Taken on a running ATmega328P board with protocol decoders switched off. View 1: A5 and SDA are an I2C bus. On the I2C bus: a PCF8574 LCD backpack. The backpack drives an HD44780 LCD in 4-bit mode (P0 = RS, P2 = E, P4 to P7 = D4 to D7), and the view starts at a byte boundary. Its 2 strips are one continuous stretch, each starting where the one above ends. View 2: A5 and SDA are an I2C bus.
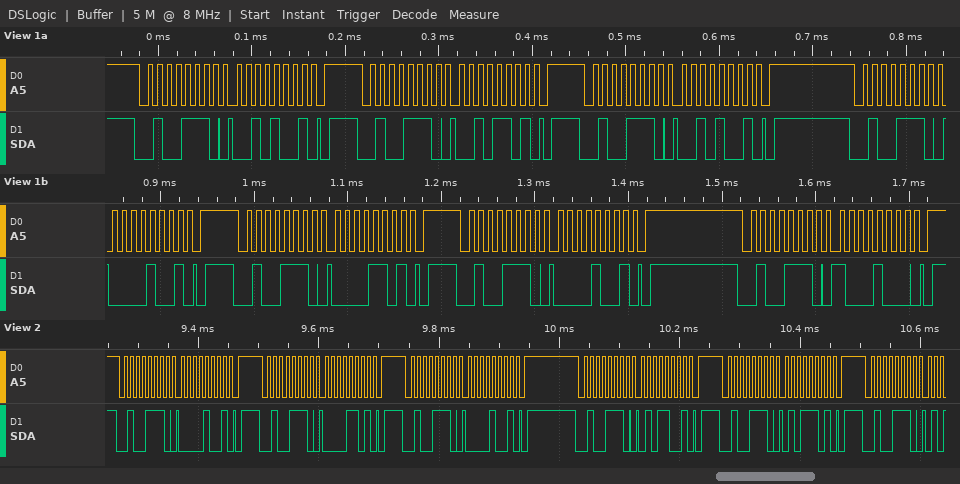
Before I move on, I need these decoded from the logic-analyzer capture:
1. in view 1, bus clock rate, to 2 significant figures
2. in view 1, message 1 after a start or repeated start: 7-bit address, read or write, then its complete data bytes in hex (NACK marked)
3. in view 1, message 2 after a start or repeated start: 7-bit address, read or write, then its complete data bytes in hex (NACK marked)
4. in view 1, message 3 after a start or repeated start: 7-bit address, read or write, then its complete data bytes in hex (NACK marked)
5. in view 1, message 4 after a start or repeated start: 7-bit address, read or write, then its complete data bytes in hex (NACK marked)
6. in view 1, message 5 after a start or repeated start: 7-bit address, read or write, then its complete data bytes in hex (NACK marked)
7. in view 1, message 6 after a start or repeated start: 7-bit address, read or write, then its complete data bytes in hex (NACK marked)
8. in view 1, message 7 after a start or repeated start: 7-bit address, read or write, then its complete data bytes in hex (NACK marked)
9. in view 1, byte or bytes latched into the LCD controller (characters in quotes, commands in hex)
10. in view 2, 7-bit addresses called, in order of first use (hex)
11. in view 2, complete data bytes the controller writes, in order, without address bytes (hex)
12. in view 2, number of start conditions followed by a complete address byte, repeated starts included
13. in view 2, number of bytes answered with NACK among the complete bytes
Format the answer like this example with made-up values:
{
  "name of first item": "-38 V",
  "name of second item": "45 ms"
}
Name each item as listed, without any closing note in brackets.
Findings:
{
  "in view 1, bus clock rate, to 2 significant figures": "100 kHz",
  "in view 1, message 1 after a start or repeated start: 7-bit address, read or write, then its complete data bytes in hex": "0x27 write: 29",
  "in view 1, message 2 after a start or repeated start: 7-bit address, read or write, then its complete data bytes in hex": "0x27 write: 2D",
  "in view 1, message 3 after a start or repeated start: 7-bit address, read or write, then its complete data bytes in hex": "0x27 write: 29",
  "in view 1, message 4 after a start or repeated start: 7-bit address, read or write, then its complete data bytes in hex": "0x27 write: 09",
  "in view 1, message 5 after a start or repeated start: 7-bit address, read or write, then its complete data bytes in hex": "0x27 write: 0D",
  "in view 1, message 6 after a start or repeated start: 7-bit address, read or write, then its complete data bytes in hex": "0x27 write: 09",
  "in view 1, message 7 after a start or repeated start: 7-bit address, read or write, then its complete data bytes in hex": "0x27 write: 88",
  "in view 1, byte or bytes latched into the LCD controller": "' '",
  "in view 2, 7-bit addresses called, in order of first use": "0x27",
  "in view 2, complete data bytes the controller writes, in order, without address bytes": "09 0D 09 59 5D",
  "in view 2, number of start conditions followed by a complete address byte, repeated starts included": "6",
  "in view 2, number of bytes answered with NACK among the complete bytes": "0"
}
